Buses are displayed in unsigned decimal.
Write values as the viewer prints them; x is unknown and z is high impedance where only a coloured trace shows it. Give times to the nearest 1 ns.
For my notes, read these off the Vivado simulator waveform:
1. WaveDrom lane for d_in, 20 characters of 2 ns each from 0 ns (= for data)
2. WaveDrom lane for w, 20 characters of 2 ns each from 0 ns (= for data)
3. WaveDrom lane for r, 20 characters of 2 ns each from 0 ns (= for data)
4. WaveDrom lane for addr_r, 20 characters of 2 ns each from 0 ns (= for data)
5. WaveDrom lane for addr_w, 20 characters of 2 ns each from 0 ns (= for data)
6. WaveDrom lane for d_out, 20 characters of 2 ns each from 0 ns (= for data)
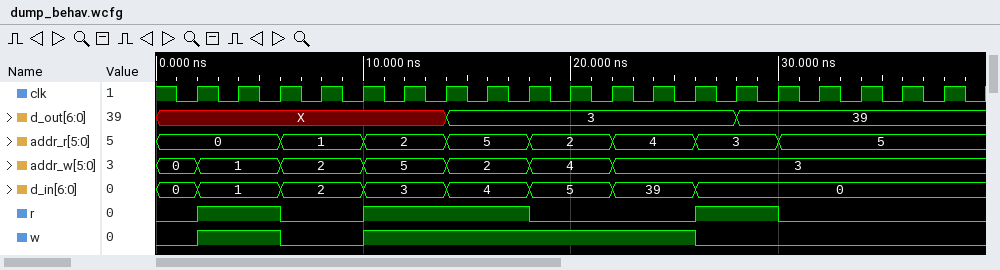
{name: 'd_in', wave: '==.=.=.=.=.=.=......', data: '0 1 2 3 4 5 39 0'}
{name: 'w', wave: '01.0.1.......0......'}
{name: 'r', wave: '01.0.1...0...1.0....'}
{name: 'addr_r', wave: '=..=.=.=.=.=.=.=....', data: '0 1 2 5 2 4 3 5'}
{name: 'addr_w', wave: '==.=.=.=.=.=........', data: '0 1 2 5 2 4 3'}
{name: 'd_out', wave: 'x......=......=.....', data: '3 39'}
